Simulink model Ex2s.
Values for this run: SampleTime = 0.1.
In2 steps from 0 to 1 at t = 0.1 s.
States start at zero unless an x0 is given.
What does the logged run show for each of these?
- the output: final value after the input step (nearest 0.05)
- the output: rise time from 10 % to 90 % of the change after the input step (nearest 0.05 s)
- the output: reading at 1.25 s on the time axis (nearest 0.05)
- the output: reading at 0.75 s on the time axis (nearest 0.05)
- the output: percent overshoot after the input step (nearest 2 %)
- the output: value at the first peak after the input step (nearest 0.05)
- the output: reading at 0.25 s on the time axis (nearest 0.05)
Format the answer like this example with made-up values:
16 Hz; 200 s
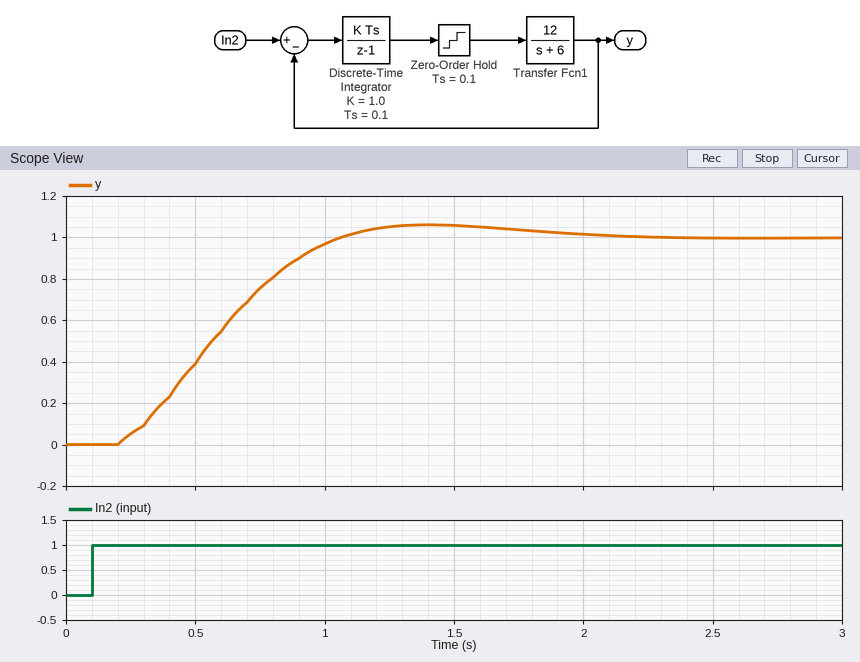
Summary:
1.00; 0.60 s; 1.05; 0.75; 6 %; 1.05; 0.05
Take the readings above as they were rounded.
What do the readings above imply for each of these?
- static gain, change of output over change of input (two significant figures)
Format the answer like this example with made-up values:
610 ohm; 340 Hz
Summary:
1.0
